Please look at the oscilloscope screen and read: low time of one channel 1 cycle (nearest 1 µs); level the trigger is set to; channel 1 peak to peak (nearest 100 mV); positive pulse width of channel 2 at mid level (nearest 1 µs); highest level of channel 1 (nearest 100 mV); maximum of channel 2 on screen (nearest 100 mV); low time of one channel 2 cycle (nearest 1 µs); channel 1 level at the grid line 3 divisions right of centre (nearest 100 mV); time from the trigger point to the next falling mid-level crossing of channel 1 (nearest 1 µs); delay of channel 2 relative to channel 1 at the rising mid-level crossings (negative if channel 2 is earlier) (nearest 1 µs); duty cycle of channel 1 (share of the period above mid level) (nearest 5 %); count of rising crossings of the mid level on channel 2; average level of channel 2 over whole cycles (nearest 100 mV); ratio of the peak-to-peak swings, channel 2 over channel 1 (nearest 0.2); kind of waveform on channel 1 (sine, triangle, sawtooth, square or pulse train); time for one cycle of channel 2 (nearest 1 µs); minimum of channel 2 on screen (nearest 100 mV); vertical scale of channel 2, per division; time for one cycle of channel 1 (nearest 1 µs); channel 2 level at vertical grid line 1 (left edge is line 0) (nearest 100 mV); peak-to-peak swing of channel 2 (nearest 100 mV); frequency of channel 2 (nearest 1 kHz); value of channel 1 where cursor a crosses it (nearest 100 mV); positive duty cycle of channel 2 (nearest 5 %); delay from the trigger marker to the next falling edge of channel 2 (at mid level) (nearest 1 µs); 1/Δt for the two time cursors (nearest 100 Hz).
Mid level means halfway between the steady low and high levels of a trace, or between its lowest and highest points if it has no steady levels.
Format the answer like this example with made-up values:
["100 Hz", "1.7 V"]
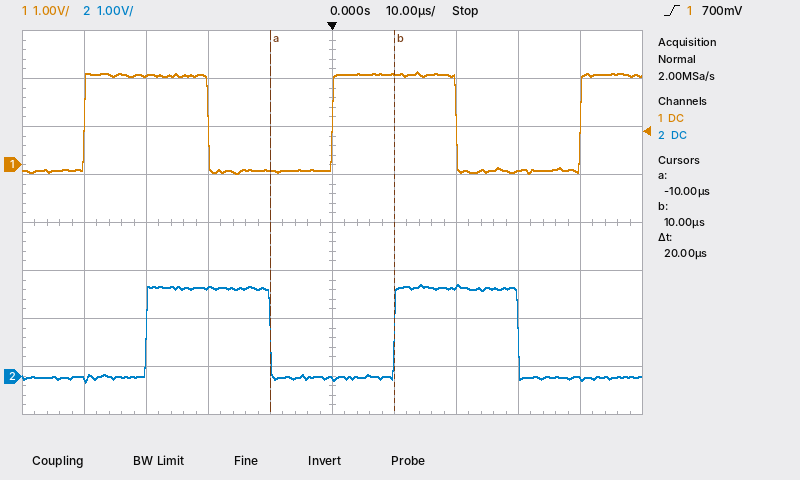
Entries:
["20 µs", "700 mV", "2.1 V", "20 µs", "1.9 V", "1.9 V", "20 µs", "-100 mV", "20 µs", "+10 µs", "50 %", "2", "900 mV", "1.0", "square", "40 µs", "-100 mV", "1 V", "40 µs", "-100 mV", "2.0 V", "25 kHz", "-100 mV", "50 %", "30 µs", "50.0 kHz"]
